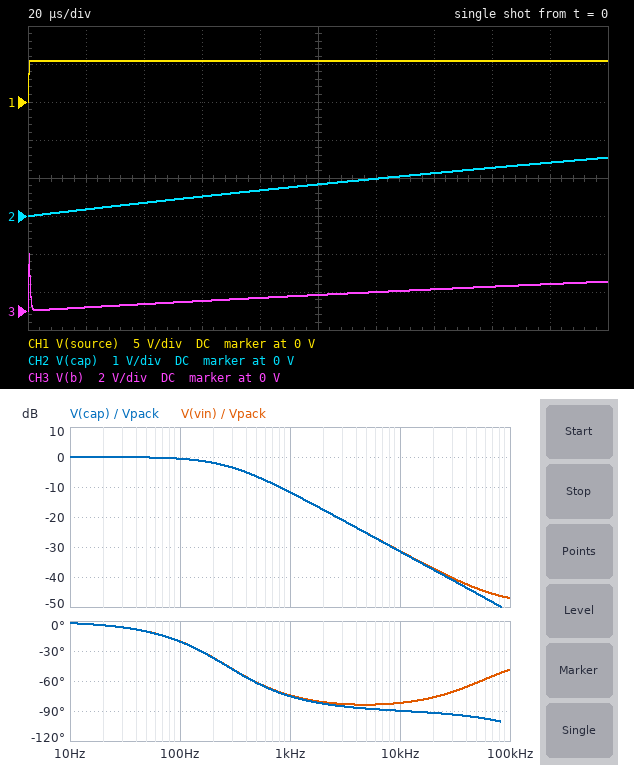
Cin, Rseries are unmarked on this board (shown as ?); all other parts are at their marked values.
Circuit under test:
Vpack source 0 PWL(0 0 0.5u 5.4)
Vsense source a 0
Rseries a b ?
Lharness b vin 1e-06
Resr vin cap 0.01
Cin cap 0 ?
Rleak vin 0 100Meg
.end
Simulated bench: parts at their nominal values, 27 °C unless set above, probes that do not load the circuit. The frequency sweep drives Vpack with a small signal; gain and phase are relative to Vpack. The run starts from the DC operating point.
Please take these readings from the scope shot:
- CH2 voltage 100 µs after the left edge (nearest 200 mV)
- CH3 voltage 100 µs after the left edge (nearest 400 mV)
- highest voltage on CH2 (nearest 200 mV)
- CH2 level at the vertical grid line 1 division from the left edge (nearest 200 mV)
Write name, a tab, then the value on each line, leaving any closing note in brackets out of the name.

CH2 voltage 100 µs after the left edge	800 mV
CH3 voltage 100 µs after the left edge	800 mV
highest voltage on CH2	1.6 V
CH2 level at the vertical grid line 1 division from the left edge	200 mV
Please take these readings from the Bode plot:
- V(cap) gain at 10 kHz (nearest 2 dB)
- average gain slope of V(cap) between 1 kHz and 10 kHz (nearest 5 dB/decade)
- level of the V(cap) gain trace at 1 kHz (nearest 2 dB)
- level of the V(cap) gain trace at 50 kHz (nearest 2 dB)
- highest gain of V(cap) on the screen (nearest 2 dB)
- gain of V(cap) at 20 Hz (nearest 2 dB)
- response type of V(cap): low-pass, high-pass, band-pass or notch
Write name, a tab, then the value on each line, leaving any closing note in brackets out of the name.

V(cap) gain at 10 kHz	-32 dB
average gain slope of V(cap) between 1 kHz and 10 kHz	-20 dB/decade
level of the V(cap) gain trace at 1 kHz	-12 dB
level of the V(cap) gain trace at 50 kHz	-46 dB
highest gain of V(cap) on the screen	0 dB
gain of V(cap) at 20 Hz	0 dB
response type of V(cap): low-pass, high-pass, band-pass or notch	low-pass
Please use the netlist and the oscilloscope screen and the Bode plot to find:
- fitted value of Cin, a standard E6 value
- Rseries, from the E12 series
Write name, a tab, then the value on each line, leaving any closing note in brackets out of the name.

fitted value of Cin, a standard E6 value	220 µF
Rseries, from the E12 series	2.7 Ω
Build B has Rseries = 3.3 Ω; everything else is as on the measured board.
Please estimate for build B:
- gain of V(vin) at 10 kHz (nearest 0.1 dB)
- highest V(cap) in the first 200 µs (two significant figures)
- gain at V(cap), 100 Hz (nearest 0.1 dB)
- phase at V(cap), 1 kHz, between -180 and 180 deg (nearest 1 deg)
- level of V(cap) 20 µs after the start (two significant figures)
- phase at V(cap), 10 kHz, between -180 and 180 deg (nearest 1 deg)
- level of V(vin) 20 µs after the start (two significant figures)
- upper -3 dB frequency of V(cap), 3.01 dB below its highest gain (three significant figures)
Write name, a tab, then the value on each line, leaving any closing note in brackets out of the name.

gain of V(vin) at 10 kHz	-33.1 dB
highest V(cap) in the first 200 µs	1.3 V
gain at V(cap), 100 Hz	-0.8 dB
phase at V(cap), 1 kHz, between -180 and 180 deg	-78 deg
level of V(cap) 20 µs after the start	140 mV
phase at V(cap), 10 kHz, between -180 and 180 deg	-90 deg
level of V(vin) 20 µs after the start	160 mV
upper -3 dB frequency of V(cap), 3.01 dB below its highest gain	219 Hz
